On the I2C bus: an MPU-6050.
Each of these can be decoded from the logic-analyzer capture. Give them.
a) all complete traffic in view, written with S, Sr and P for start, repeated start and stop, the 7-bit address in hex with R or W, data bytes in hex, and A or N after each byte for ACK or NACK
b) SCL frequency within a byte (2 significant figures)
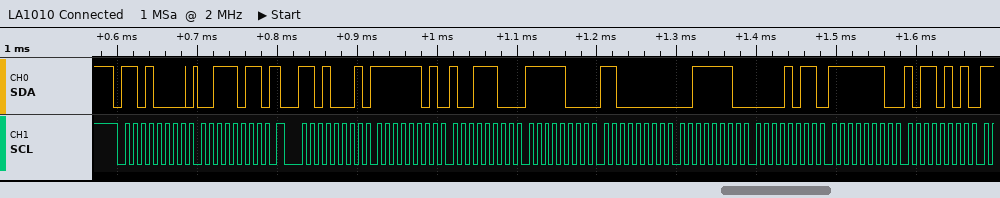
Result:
S 68W A 3B A Sr 68R A FD A 9C A F8 A C0 A 3E A 0B A FE A B5 A
100 kHz
